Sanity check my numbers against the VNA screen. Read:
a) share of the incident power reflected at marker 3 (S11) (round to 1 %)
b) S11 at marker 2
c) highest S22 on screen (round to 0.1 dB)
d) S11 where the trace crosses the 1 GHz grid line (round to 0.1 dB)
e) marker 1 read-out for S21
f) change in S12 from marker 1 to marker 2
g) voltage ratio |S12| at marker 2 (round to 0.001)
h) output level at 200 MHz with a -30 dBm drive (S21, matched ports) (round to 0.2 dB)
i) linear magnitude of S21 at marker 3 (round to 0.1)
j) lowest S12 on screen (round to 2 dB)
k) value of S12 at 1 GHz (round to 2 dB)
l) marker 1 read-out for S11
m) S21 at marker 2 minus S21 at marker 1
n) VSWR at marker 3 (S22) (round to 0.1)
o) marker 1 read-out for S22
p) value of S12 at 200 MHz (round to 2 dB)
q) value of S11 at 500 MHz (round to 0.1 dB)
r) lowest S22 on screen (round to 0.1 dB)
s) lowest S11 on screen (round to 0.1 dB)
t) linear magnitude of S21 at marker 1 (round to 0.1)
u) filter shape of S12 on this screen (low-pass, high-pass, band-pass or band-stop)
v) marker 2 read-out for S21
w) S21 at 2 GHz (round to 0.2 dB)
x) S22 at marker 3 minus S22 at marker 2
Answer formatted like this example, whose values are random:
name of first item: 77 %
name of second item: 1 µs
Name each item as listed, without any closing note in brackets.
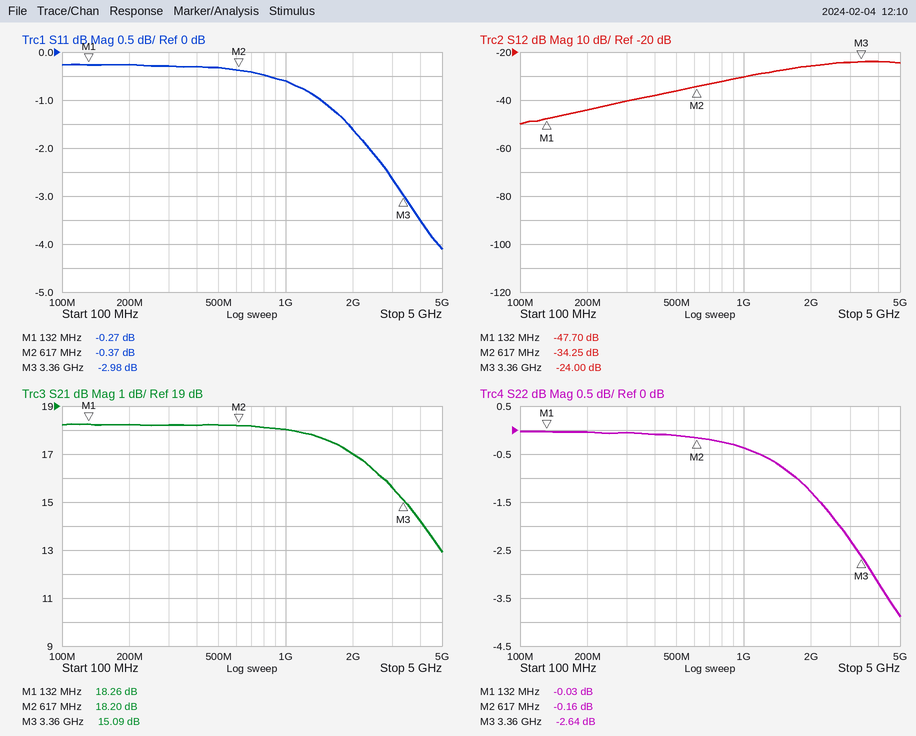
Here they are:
share of the incident power reflected at marker 3 (S11): 50 %
S11 at marker 2: -0.37 dB
highest S22 on screen: 0.0 dB
S11 where the trace crosses the 1 GHz grid line: -0.6 dB
marker 1 read-out for S21: 18.26 dB
change in S12 from marker 1 to marker 2: 13.45 dB
voltage ratio |S12| at marker 2: 0.019
output level at 200 MHz with a -30 dBm drive (S21, matched ports): -11.8 dBm
linear magnitude of S21 at marker 3: 5.7
lowest S12 on screen: -50 dB
value of S12 at 1 GHz: -30 dB
marker 1 read-out for S11: -0.27 dB
S21 at marker 2 minus S21 at marker 1: -0.06 dB
VSWR at marker 3 (S22): 6.6
marker 1 read-out for S22: -0.03 dB
value of S12 at 200 MHz: -44 dB
value of S11 at 500 MHz: -0.3 dB
lowest S22 on screen: -3.9 dB
lowest S11 on screen: -4.1 dB
linear magnitude of S21 at marker 1: 8.2
filter shape of S12 on this screen: high-pass
marker 2 read-out for S21: 18.20 dB
S21 at 2 GHz: 17.0 dB
S22 at marker 3 minus S22 at marker 2: -2.48 dB
